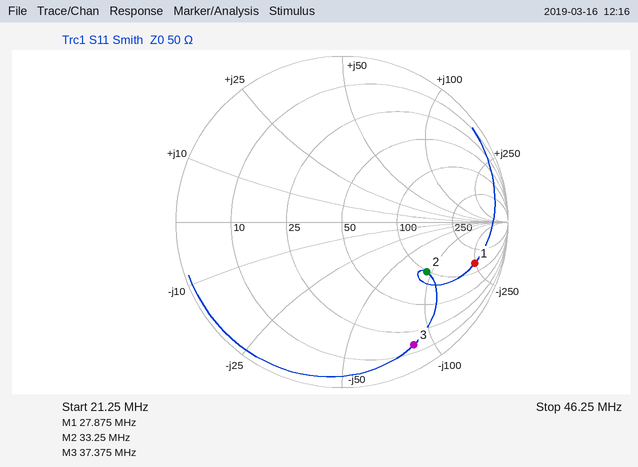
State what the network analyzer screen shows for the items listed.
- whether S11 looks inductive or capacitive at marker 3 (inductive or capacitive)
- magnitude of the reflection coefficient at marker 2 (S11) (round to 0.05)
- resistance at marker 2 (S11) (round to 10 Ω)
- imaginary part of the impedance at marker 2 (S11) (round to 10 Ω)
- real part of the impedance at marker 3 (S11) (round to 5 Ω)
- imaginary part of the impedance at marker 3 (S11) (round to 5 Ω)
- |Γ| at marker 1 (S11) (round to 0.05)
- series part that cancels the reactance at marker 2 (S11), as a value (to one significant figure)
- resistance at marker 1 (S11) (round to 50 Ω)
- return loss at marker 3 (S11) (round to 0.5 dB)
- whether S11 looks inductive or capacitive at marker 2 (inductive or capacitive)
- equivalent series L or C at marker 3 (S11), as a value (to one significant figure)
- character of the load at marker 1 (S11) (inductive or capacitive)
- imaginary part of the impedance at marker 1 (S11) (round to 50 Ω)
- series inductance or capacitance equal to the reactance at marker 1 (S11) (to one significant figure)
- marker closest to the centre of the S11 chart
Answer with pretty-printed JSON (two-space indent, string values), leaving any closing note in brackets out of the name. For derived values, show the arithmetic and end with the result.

{
  "whether S11 looks inductive or capacitive at marker 3": "capacitive",
  "magnitude of the reflection coefficient at marker 2 (S11)": "0.60",
  "resistance at marker 2 (S11)": "100 Ω",
  "imaginary part of the impedance at marker 2 (S11)": "-90 Ω",
  "real part of the impedance at marker 3 (S11)": "15 Ω",
  "imaginary part of the impedance at marker 3 (S11)": "-85 Ω",
  "|Γ| at marker 1 (S11)": "0.85",
  "series part that cancels the reactance at marker 2 (S11), as a value": "L = 90 Ω/(2π × 33.25 MHz) ≈ 431 nH, so 400 nH to one significant figure",
  "resistance at marker 1 (S11)": "150 Ω",
  "return loss at marker 3 (S11)": "1.5 dB",
  "whether S11 looks inductive or capacitive at marker 2": "capacitive",
  "equivalent series L or C at marker 3 (S11), as a value": "C = 1/(2π × 37.375 MHz × 85 Ω) ≈ 50 pF",
  "character of the load at marker 1 (S11)": "capacitive",
  "imaginary part of the impedance at marker 1 (S11)": "-250 Ω",
  "series inductance or capacitance equal to the reactance at marker 1 (S11)": "C = 1/(2π × 27.875 MHz × 250 Ω) ≈ 22.8 pF, so 20 pF to one significant figure",
  "marker closest to the centre of the S11 chart": "marker 2"
}
